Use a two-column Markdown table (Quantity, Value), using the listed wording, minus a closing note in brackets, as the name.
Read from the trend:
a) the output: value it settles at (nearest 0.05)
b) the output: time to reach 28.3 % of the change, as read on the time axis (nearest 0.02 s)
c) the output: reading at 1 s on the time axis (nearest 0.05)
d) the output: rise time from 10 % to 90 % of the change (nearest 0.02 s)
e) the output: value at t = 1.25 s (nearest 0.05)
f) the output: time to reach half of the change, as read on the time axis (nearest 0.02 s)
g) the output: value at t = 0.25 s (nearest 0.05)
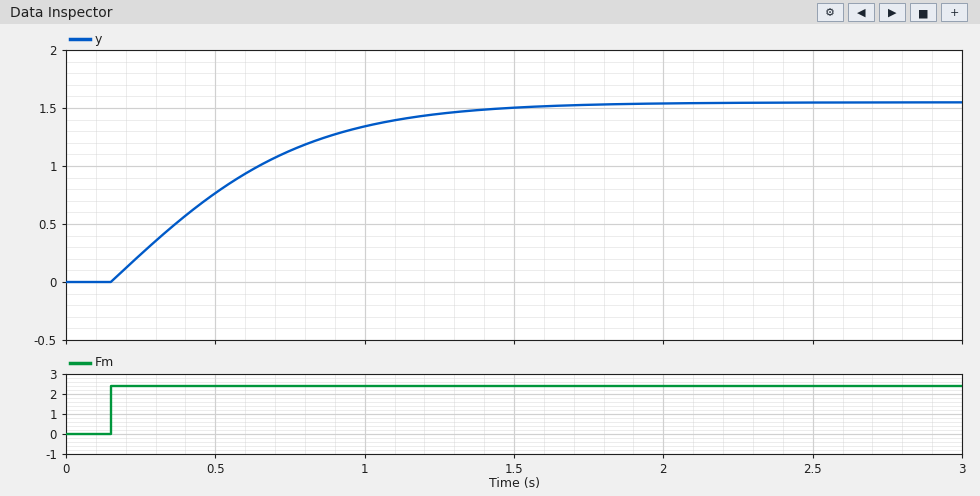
| Quantity | Value |
|---|---|
| the output: value it settles at | 1.55 |
| the output: time to reach 28.3 % of the change, as read on the time axis | 0.34 s |
| the output: reading at 1 s on the time axis | 1.35 |
| the output: rise time from 10 % to 90 % of the change | 0.88 s |
| the output: value at t = 1.25 s | 1.45 |
| the output: time to reach half of the change, as read on the time axis | 0.50 s |
| the output: value at t = 0.25 s | 0.25 |
